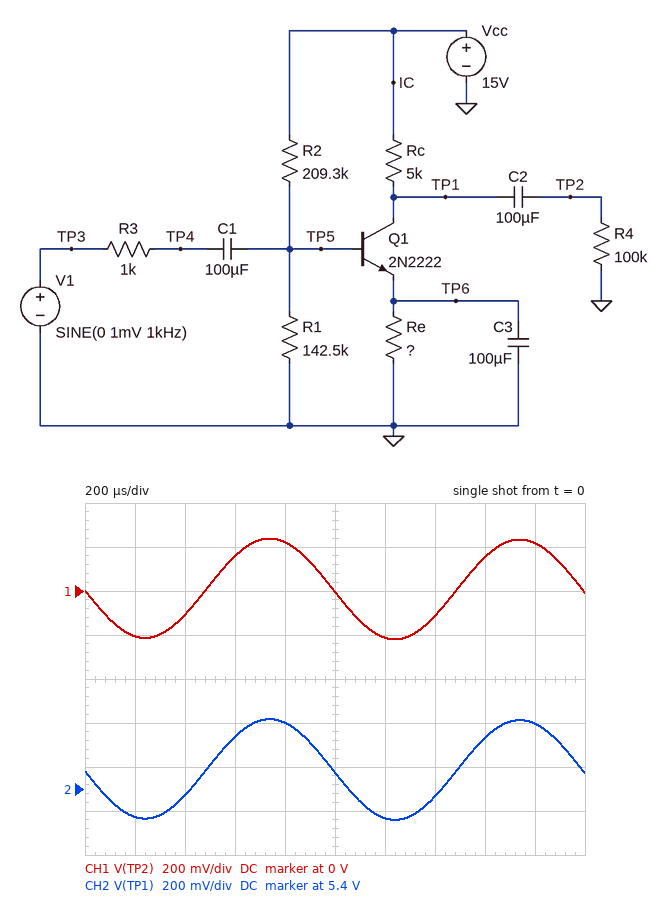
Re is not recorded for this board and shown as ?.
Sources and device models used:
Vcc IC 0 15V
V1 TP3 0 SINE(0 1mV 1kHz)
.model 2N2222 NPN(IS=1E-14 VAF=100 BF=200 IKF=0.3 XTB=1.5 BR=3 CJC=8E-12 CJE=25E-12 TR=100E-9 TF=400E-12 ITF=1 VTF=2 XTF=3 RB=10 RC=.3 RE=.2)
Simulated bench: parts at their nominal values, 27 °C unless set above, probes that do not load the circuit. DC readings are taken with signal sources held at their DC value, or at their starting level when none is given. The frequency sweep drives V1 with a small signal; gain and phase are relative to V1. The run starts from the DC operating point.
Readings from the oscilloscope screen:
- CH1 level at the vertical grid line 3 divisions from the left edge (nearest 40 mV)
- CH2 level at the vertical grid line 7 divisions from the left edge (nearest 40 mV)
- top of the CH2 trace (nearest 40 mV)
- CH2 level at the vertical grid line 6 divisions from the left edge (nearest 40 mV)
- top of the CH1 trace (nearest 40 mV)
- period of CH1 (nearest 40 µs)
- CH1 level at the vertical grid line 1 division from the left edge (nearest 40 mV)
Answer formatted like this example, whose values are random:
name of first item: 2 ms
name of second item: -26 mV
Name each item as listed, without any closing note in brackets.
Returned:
CH1 level at the vertical grid line 3 divisions from the left edge: 160 mV
CH2 level at the vertical grid line 7 divisions from the left edge: 5.36 V
top of the CH2 trace: 5.72 V
CH2 level at the vertical grid line 6 divisions from the left edge: 5.28 V
top of the CH1 trace: 240 mV
period of CH1: 1.00 ms
CH1 level at the vertical grid line 1 division from the left edge: -200 mV
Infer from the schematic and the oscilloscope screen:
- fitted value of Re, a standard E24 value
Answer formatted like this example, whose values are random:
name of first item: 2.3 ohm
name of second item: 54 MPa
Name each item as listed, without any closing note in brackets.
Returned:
fitted value of Re, a standard E24 value: 2.4 kΩ
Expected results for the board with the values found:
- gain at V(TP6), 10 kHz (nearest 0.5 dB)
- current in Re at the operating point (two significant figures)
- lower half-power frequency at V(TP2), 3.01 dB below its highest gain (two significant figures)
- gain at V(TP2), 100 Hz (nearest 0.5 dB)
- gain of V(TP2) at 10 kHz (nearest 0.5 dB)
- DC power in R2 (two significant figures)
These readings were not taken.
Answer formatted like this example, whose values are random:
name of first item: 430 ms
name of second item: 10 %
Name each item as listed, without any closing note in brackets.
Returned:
gain at V(TP6), 10 kHz: -42.5 dB
current in Re at the operating point: 1.9 mA
lower half-power frequency at V(TP2), 3.01 dB below its highest gain: 79 Hz
gain at V(TP2), 100 Hz: 45.0 dB
gain of V(TP2) at 10 kHz: 47.0 dB
DC power in R2: 450 µW
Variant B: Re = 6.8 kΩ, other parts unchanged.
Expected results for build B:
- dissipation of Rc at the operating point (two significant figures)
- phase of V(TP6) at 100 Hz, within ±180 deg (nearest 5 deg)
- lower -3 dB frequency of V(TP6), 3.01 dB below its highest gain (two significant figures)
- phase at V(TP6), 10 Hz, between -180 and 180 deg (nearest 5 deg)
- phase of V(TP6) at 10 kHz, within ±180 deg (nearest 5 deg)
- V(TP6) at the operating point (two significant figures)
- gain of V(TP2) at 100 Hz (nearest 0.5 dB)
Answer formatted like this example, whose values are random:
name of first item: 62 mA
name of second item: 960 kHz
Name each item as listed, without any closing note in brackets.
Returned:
dissipation of Rc at the operating point: 2.8 mW
phase of V(TP6) at 100 Hz, within ±180 deg: -70 deg
lower -3 dB frequency of V(TP6), 3.01 dB below its highest gain: 20 mHz
phase at V(TP6), 10 Hz, between -180 and 180 deg: -15 deg
phase of V(TP6) at 10 kHz, within ±180 deg: -90 deg
V(TP6) at the operating point: 5.1 V
gain of V(TP2) at 100 Hz: 40.5 dB
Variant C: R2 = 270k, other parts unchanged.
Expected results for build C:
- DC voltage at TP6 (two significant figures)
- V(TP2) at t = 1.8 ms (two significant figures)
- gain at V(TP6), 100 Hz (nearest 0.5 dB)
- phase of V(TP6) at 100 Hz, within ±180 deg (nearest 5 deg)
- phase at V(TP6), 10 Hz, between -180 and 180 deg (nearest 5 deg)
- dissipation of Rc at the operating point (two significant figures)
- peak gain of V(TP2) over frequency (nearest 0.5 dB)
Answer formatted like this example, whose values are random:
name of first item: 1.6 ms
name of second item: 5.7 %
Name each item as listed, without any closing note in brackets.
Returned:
DC voltage at TP6: 3.8 V
V(TP2) at t = 1.8 ms: 190 mV
gain at V(TP6), 100 Hz: -5.0 dB
phase of V(TP6) at 100 Hz, within ±180 deg: -55 deg
phase at V(TP6), 10 Hz, between -180 and 180 deg: -10 deg
dissipation of Rc at the operating point: 12 mW
peak gain of V(TP2) over frequency: 46.0 dB
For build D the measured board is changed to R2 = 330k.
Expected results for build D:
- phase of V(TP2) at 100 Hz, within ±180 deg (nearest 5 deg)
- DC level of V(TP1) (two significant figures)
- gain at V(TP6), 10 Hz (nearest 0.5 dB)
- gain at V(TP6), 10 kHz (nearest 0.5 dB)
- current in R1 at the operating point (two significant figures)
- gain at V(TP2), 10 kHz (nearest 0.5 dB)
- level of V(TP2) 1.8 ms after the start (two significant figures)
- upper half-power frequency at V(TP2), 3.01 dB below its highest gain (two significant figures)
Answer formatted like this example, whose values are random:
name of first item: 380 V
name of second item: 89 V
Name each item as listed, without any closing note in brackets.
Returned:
phase of V(TP2) at 100 Hz, within ±180 deg: -150 deg
DC level of V(TP1): 8.3 V
gain at V(TP6), 10 Hz: -0.5 dB
gain at V(TP6), 10 kHz: -44.5 dB
current in R1 at the operating point: 27 µA
gain at V(TP2), 10 kHz: 45.0 dB
level of V(TP2) 1.8 ms after the start: 170 mV
upper half-power frequency at V(TP2), 3.01 dB below its highest gain: 190 kHz
